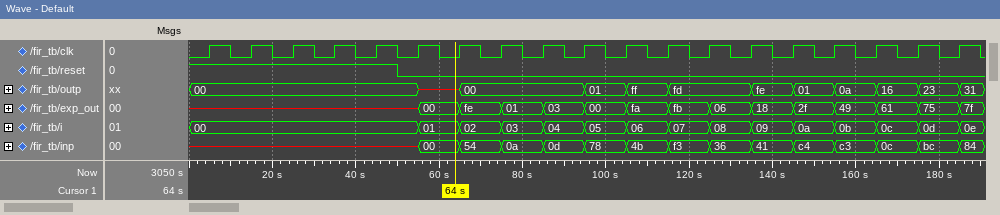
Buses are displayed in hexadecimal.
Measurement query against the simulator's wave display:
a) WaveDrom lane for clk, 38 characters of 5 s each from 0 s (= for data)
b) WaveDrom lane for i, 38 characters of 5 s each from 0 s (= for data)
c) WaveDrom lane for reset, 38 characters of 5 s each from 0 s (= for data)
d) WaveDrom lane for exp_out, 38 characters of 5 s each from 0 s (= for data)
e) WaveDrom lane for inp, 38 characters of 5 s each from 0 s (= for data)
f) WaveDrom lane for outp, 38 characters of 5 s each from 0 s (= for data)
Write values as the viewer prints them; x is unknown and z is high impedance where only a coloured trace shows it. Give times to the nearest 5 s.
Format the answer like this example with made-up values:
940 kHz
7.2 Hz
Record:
{name: 'clk', wave: '01010101010101010101010101010101010101'}
{name: 'i', wave: '=..........=.=.=.=.=.=.=.=.=.=.=.=.=.=', data: '00 01 02 03 04 05 06 07 08 09 0a 0b 0c 0d 0e'}
{name: 'reset', wave: '1.........0...........................'}
{name: 'exp_out', wave: 'x..........=.=.=.=.=.=.=.=.=.=.=.=.=.=', data: '00 fe 01 03 00 fa fb 06 18 2f 49 61 75 7f'}
{name: 'inp', wave: 'x..........=.=.=.=.=.=.=.=.=.=.=.=.=.=', data: '00 54 0a 0d 78 4b f3 36 41 c4 c3 0c bc 84'}
{name: 'outp', wave: '=..........x.=.....=.=.=...=.=.=.=.=.=', data: '00 00 01 ff fd fe 01 0a 16 23 31'}
